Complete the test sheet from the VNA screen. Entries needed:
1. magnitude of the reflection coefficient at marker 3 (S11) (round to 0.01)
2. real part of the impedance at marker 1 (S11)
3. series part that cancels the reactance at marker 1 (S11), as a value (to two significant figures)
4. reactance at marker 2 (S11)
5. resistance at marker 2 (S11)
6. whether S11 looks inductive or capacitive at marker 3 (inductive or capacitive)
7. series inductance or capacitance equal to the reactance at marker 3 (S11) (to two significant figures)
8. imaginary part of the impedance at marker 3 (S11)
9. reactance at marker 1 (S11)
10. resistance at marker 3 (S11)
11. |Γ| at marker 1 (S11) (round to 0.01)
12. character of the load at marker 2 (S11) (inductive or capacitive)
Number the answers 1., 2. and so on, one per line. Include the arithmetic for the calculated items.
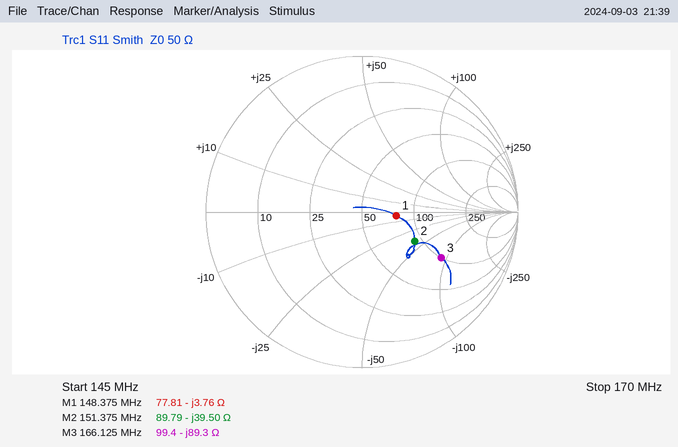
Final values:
1. 0.59
2. 77.81 Ω
3. L = 3.76 Ω/(2π × 148.375 MHz) ≈ 4.0 nH
4. -39.50 Ω
5. 89.79 Ω
6. capacitive
7. C = 1/(2π × 166.125 MHz × 89.3 Ω) ≈ 11 pF
8. -89.3 Ω
9. -3.76 Ω
10. 99.4 Ω
11. 0.22
12. capacitive
